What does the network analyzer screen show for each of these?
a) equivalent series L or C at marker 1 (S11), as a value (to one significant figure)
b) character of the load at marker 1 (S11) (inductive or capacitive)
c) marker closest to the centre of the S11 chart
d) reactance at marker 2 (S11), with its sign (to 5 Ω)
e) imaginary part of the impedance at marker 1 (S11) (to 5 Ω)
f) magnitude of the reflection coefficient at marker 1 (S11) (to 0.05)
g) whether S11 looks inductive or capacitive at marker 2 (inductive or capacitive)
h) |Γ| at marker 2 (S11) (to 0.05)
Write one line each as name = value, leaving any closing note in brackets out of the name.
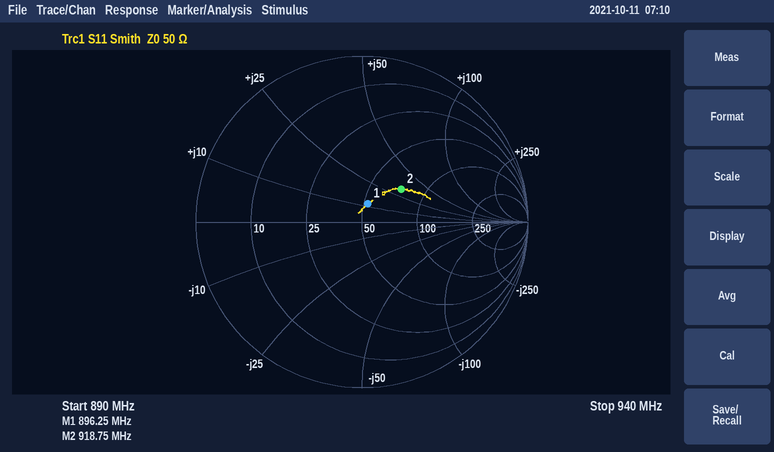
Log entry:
equivalent series L or C at marker 1 (S11), as a value = 2 nH
character of the load at marker 1 (S11) = inductive
marker closest to the centre of the S11 chart = marker 1
reactance at marker 2 (S11), with its sign = +30 Ω
imaginary part of the impedance at marker 1 (S11) = +10 Ω
magnitude of the reflection coefficient at marker 1 (S11) = 0.10
whether S11 looks inductive or capacitive at marker 2 = inductive
|Γ| at marker 2 (S11) = 0.30
